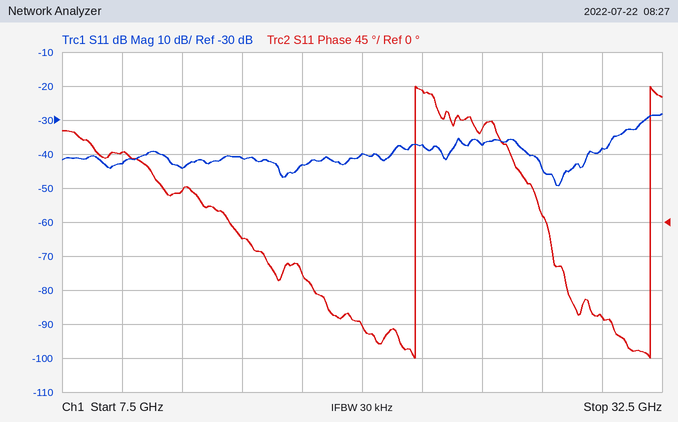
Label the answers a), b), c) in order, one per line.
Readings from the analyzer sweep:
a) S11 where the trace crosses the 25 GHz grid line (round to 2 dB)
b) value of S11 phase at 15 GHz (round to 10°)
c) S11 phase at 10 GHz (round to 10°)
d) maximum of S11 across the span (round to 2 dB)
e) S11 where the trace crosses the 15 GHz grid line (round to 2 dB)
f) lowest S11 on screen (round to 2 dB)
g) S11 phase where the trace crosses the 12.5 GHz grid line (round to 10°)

a) -38 dB
b) -20°
c) 90°
d) -28 dB
e) -42 dB
f) -50 dB
g) 40°
